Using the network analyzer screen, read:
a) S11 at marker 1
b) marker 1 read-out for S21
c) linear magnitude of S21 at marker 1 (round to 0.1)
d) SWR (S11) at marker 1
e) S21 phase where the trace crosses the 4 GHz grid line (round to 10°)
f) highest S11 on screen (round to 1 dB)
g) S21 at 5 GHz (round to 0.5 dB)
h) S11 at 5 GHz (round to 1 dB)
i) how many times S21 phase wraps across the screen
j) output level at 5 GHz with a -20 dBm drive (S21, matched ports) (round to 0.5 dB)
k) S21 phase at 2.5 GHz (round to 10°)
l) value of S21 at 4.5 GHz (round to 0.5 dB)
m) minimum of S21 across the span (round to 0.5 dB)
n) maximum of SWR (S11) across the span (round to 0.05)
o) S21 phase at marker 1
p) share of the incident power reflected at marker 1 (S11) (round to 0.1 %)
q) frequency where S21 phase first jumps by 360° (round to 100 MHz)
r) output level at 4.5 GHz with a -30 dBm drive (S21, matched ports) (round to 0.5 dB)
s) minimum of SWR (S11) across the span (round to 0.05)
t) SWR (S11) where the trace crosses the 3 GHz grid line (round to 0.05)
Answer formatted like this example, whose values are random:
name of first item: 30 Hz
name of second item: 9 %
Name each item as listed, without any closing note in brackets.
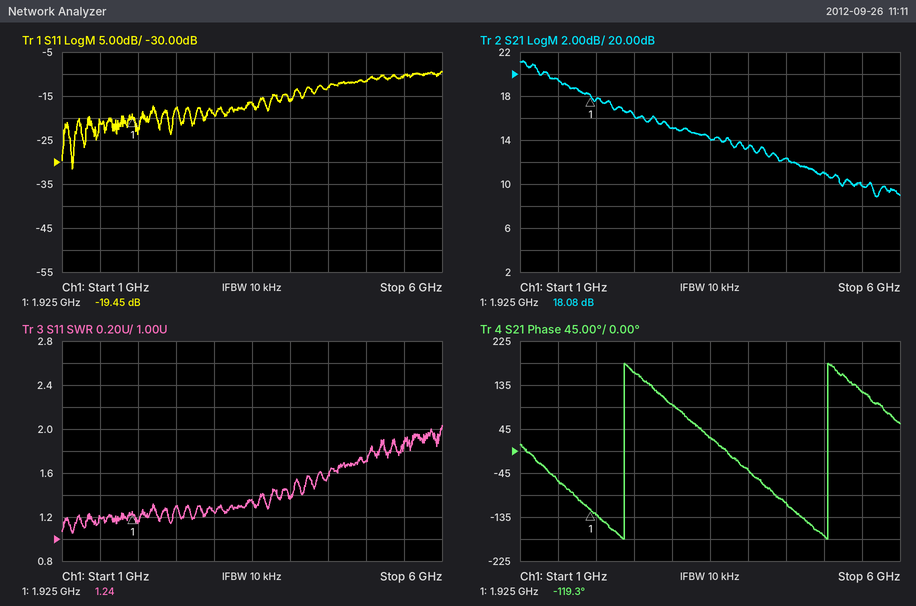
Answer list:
S11 at marker 1: -19.45 dB
marker 1 read-out for S21: 18.08 dB
linear magnitude of S21 at marker 1: 8.0
SWR (S11) at marker 1: 1.24
S21 phase where the trace crosses the 4 GHz grid line: -40°
highest S11 on screen: -9 dB
S21 at 5 GHz: 11.0 dB
S11 at 5 GHz: -12 dB
how many times S21 phase wraps across the screen: 2
output level at 5 GHz with a -20 dBm drive (S21, matched ports): -9.0 dBm
S21 phase at 2.5 GHz: 160°
value of S21 at 4.5 GHz: 12.5 dB
minimum of S21 across the span: 9.0 dB
maximum of SWR (S11) across the span: 2.05
S21 phase at marker 1: -119.3°
share of the incident power reflected at marker 1 (S11): 1.1 %
frequency where S21 phase first jumps by 360°: 2.4 GHz
output level at 4.5 GHz with a -30 dBm drive (S21, matched ports): -17.5 dBm
minimum of SWR (S11) across the span: 1.05
SWR (S11) where the trace crosses the 3 GHz grid line: 1.25
